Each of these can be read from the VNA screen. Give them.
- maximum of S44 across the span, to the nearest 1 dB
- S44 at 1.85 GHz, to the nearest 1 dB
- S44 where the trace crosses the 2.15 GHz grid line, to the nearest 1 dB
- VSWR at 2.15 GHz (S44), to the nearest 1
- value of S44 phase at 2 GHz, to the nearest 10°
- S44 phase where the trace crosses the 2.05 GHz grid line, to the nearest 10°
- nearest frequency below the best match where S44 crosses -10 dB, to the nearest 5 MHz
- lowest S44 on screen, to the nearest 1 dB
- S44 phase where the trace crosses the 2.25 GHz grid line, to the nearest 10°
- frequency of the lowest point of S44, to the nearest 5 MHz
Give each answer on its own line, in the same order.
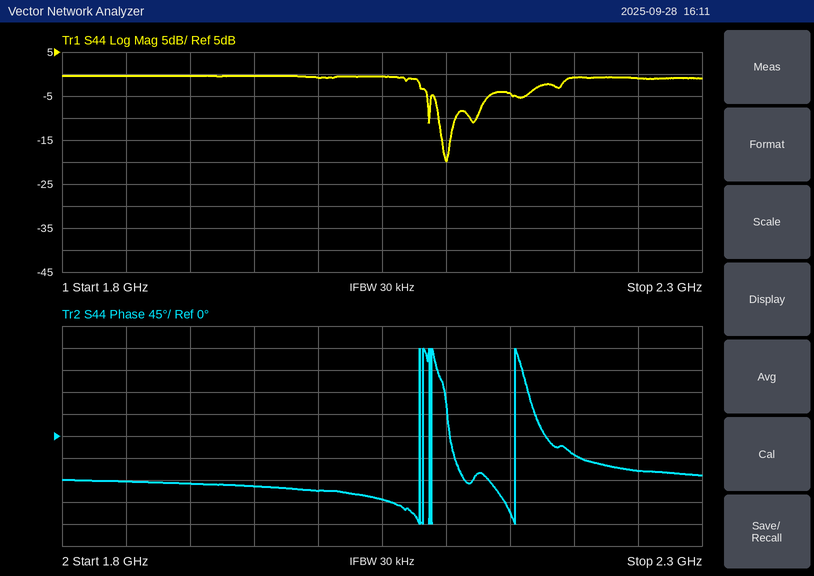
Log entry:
0 dB
0 dB
-4 dB
4
-110°
-130°
2.095 GHz
-20 dB
-70°
2.100 GHz
